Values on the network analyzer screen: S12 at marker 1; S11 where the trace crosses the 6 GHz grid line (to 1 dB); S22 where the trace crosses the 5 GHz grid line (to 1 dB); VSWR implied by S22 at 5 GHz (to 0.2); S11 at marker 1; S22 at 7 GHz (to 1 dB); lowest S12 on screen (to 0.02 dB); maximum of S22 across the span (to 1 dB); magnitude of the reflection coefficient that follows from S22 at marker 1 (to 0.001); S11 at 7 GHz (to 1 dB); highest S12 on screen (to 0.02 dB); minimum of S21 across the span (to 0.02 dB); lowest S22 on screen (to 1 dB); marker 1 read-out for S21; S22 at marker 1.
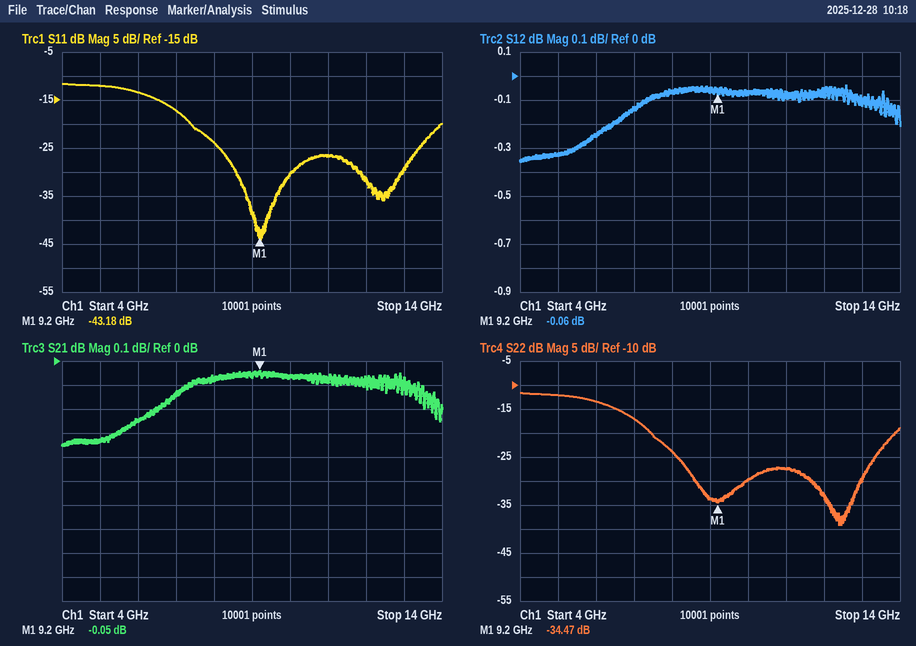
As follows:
-0.06 dB
-13 dB
-12 dB
1.6
-43.18 dB
-17 dB
-0.36 dB
-12 dB
0.019
-17 dB
-0.04 dB
-0.36 dB
-39 dB
-0.05 dB
-34.47 dB
